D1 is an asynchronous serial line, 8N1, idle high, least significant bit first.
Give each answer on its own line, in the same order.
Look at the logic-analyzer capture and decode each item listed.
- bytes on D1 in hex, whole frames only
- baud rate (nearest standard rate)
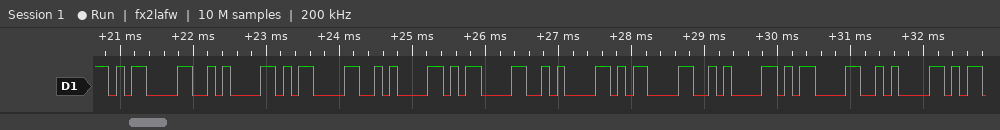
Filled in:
0x0D 0x0A 0x0D 0x0A 0x0D 0x0A 0x0D 0x0A 0x0D 0x0A
9600 baud
